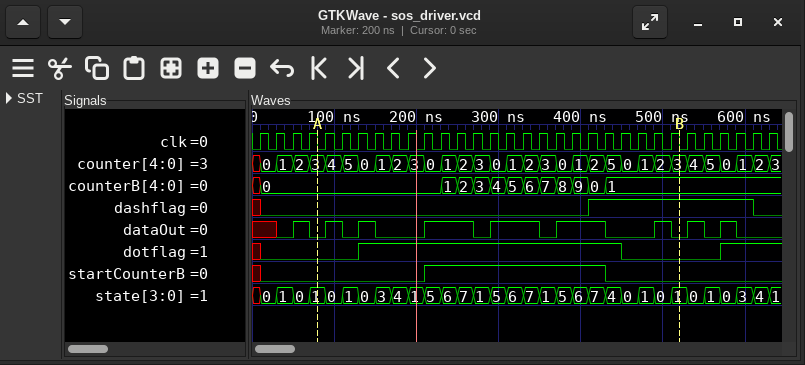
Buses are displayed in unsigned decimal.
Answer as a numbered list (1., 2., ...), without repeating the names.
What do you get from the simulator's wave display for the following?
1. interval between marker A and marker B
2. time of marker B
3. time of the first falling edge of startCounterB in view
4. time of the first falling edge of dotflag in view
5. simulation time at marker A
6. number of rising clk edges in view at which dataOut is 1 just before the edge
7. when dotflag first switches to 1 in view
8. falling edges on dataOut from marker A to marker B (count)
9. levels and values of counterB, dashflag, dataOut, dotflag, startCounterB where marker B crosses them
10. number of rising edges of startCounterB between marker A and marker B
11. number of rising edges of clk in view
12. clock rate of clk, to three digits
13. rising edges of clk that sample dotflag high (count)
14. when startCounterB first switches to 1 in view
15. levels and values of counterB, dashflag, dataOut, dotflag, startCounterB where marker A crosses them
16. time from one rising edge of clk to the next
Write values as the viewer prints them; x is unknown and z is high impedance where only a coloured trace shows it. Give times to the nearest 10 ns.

1. 440 ns
2. 520 ns
3. 430 ns
4. 450 ns
5. 80 ns
6. 15
7. 130 ns
8. 6
9. counterB=1, dashflag=1, dataOut=0, dotflag=0, startCounterB=0
10. 1
11. 32
12. 50.0 MHz
13. 19
14. 210 ns
15. counterB=0, dashflag=0, dataOut=0, dotflag=0, startCounterB=0
16. 20 ns
